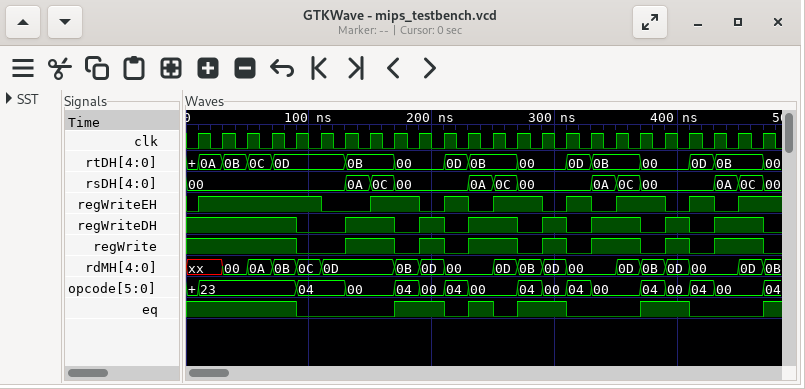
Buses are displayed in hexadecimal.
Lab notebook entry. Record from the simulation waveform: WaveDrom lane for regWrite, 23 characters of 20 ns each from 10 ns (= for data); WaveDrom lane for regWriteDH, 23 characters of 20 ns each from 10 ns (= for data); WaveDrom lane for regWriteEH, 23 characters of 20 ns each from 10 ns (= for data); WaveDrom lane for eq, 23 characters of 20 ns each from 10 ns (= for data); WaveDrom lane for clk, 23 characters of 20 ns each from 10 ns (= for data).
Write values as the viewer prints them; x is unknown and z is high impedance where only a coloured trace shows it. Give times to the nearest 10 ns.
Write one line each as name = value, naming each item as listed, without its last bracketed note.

WaveDrom lane for regWrite, 23 characters of 20 ns each from 10 ns = {name: 'regWrite', wave: '1...0.1.0101.0101.0101.'}
WaveDrom lane for regWriteDH, 23 characters of 20 ns each from 10 ns = {name: 'regWriteDH', wave: '1...0.1.0101.0101.0101.'}
WaveDrom lane for regWriteEH, 23 characters of 20 ns each from 10 ns = {name: 'regWriteEH', wave: '1....0.1.0101.0101.0101'}
WaveDrom lane for eq, 23 characters of 20 ns each from 10 ns = {name: 'eq', wave: '1...0...1.0101.0..1.0..'}
WaveDrom lane for clk, 23 characters of 20 ns each from 10 ns = {name: 'clk', wave: 'p......................'}
